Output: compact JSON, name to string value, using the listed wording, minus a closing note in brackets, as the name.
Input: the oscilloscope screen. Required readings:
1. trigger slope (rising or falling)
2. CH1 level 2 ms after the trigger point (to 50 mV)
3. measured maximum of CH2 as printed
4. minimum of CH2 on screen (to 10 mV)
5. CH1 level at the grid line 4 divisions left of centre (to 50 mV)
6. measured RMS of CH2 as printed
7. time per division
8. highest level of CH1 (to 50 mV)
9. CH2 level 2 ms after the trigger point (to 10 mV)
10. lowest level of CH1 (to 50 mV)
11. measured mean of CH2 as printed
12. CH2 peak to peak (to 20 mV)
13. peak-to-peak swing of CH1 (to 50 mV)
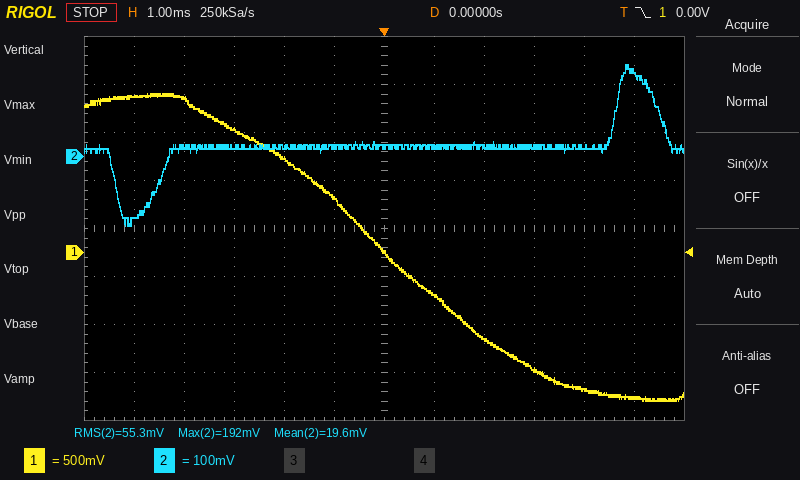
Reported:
{"trigger slope": "falling", "CH1 level 2 ms after the trigger point": "-900 mV", "measured maximum of CH2 as printed": "192 mV", "minimum of CH2 on screen": "-140 mV", "CH1 level at the grid line 4 divisions left of centre": "1.60 V", "measured RMS of CH2 as printed": "55.3 mV", "time per division": "1 ms", "highest level of CH1": "1.65 V", "CH2 level 2 ms after the trigger point": "20 mV", "lowest level of CH1": "-1.55 V", "measured mean of CH2 as printed": "19.6 mV", "CH2 peak to peak": "340 mV", "peak-to-peak swing of CH1": "3.20 V"}
